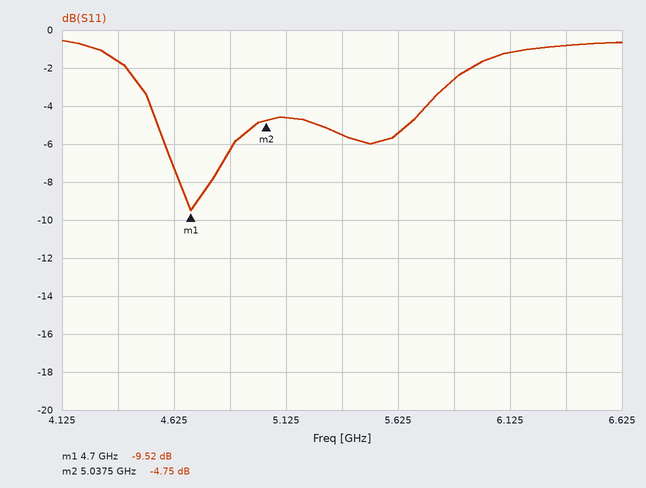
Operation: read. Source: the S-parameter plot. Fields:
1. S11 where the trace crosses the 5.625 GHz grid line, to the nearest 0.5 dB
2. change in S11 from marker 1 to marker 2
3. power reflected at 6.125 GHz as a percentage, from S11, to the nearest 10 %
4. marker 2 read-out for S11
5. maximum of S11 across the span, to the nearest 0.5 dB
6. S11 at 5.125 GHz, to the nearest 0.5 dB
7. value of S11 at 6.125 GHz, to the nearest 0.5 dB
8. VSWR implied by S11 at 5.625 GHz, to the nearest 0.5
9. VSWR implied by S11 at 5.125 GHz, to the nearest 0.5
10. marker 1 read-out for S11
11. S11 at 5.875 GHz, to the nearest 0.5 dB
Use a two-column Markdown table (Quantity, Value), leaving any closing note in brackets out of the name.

| Quantity | Value |
|---|---|
| S11 where the trace crosses the 5.625 GHz grid line, to the nearest 0.5 dB | -5.5 dB |
| change in S11 from marker 1 to marker 2 | 4.77 dB |
| power reflected at 6.125 GHz as a percentage, from S11, to the nearest 10 % | 80 % |
| marker 2 read-out for S11 | -4.75 dB |
| maximum of S11 across the span, to the nearest 0.5 dB | -0.5 dB |
| S11 at 5.125 GHz, to the nearest 0.5 dB | -4.5 dB |
| value of S11 at 6.125 GHz, to the nearest 0.5 dB | -1.0 dB |
| VSWR implied by S11 at 5.625 GHz, to the nearest 0.5 | 3.5 |
| VSWR implied by S11 at 5.125 GHz, to the nearest 0.5 | 4.0 |
| marker 1 read-out for S11 | -9.52 dB |
| S11 at 5.875 GHz, to the nearest 0.5 dB | -2.5 dB |
